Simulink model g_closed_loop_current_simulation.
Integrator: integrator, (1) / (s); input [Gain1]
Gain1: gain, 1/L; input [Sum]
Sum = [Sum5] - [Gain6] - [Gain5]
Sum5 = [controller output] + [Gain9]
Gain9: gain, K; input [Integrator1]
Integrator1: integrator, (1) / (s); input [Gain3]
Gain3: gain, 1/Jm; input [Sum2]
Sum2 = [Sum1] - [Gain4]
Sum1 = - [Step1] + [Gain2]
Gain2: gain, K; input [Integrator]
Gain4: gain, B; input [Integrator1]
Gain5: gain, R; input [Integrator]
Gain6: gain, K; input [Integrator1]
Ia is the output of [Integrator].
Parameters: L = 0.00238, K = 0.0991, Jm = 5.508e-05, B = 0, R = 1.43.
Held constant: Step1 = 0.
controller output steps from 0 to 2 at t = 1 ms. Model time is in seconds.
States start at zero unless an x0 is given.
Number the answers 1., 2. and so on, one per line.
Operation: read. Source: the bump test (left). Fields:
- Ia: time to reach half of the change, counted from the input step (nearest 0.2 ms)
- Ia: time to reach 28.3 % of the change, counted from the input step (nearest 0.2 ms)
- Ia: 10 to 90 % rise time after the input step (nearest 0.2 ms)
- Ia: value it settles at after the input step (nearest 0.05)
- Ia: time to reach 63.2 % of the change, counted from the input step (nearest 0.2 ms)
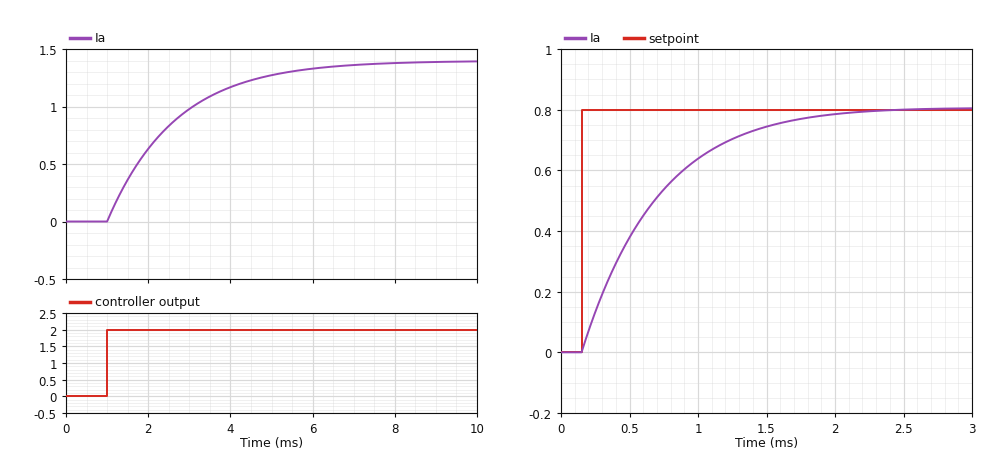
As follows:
1. 1.2 ms
2. 0.6 ms
3. 3.6 ms
4. 1.40
5. 1.6 ms
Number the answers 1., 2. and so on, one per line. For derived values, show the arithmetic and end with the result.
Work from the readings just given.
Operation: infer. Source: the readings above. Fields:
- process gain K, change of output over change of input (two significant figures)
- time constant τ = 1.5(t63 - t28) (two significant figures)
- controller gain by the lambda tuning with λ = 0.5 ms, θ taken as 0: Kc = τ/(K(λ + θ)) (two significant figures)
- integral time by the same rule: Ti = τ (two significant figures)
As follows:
1. (1.4 - 0) / 2 = 0.70
2. 1.5 × (1.6 - 0.6) = 1.5 ms
3. 1.5 / (0.7 × (0.5 + 0)) = 4.3
4. 1.5 ms
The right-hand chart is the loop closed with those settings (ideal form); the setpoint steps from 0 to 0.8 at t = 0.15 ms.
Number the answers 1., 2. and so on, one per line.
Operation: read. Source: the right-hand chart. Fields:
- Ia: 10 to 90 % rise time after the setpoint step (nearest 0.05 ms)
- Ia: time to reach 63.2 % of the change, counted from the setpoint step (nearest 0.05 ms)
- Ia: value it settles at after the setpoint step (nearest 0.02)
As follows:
1. 1.15 ms
2. 0.55 ms
3. 0.80
